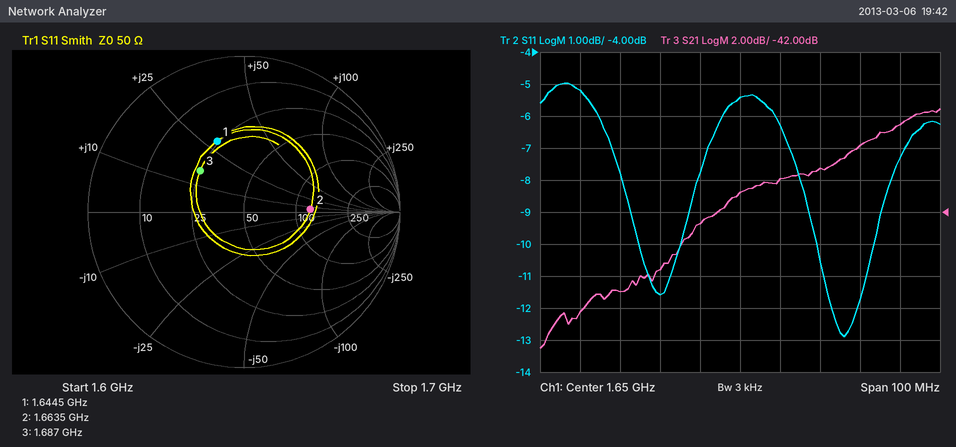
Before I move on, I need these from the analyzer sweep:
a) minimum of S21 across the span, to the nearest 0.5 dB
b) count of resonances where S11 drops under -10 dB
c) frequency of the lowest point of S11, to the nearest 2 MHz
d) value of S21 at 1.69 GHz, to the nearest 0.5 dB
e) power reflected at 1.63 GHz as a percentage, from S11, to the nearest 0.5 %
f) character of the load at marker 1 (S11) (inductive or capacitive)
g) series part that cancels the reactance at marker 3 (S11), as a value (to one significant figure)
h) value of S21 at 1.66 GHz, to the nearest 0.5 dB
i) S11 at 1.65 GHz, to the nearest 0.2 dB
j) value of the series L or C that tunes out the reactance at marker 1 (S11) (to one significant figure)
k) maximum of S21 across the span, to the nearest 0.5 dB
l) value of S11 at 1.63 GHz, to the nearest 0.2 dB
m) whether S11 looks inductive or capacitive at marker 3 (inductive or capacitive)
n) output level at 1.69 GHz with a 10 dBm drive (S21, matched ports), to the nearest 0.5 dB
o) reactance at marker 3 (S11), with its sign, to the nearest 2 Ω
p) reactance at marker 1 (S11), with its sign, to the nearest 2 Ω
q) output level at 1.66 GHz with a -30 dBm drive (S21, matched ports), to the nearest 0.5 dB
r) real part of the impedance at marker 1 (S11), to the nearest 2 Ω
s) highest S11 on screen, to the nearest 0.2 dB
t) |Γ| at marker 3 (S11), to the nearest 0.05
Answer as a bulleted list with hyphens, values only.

- -50.5 dB
- 2
- 1.676 GHz
- -36.5 dB
- 7.0 %
- inductive
- 6 pF
- -40.0 dB
- -5.4 dB
- 3 pF
- -35.5 dB
- -11.6 dB
- inductive
- -26.5 dBm
- +16 Ω
- +28 Ω
- -70.0 dBm
- 24 Ω
- -5.0 dB
- 0.40
